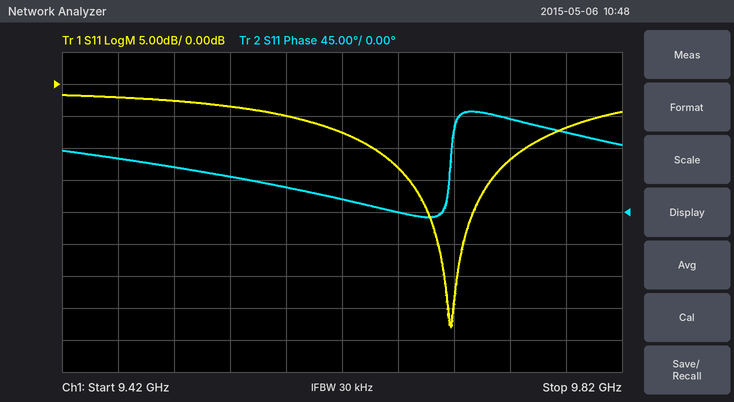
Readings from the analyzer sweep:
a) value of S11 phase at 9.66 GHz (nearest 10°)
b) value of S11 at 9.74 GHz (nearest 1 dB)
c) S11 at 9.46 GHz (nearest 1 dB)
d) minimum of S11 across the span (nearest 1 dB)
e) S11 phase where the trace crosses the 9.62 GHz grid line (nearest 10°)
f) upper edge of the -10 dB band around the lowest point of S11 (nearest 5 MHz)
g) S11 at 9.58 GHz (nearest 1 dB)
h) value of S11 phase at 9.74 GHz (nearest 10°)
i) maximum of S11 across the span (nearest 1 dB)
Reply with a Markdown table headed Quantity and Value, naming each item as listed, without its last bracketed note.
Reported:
| Quantity | Value |
|---|---|
| value of S11 phase at 9.66 GHz | 0° |
| value of S11 at 9.74 GHz | -12 dB |
| S11 at 9.46 GHz | -2 dB |
| minimum of S11 across the span | -38 dB |
| S11 phase where the trace crosses the 9.62 GHz grid line | 20° |
| upper edge of the -10 dB band around the lowest point of S11 | 9.750 GHz |
| S11 at 9.58 GHz | -5 dB |
| value of S11 phase at 9.74 GHz | 130° |
| maximum of S11 across the span | -2 dB |
